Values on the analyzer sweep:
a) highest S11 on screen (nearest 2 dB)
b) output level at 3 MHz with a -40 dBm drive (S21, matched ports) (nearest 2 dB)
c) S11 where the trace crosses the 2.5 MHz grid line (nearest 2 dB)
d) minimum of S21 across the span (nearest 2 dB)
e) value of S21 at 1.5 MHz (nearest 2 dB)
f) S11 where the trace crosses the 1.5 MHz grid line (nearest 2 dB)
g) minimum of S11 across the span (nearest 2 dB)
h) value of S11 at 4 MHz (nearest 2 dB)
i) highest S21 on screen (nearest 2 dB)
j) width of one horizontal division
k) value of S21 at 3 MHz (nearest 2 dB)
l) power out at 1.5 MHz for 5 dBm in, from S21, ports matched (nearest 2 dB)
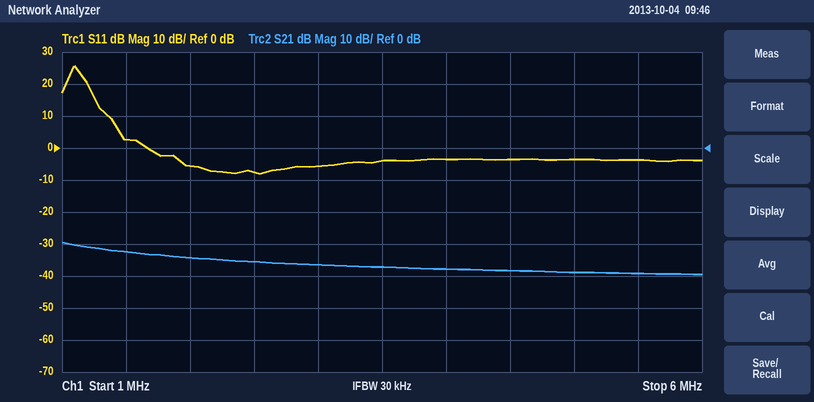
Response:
26 dB
-76 dBm
-8 dB
-40 dB
-32 dB
2 dB
-8 dB
-4 dB
-30 dB
500 kHz
-36 dB
-28 dBm
